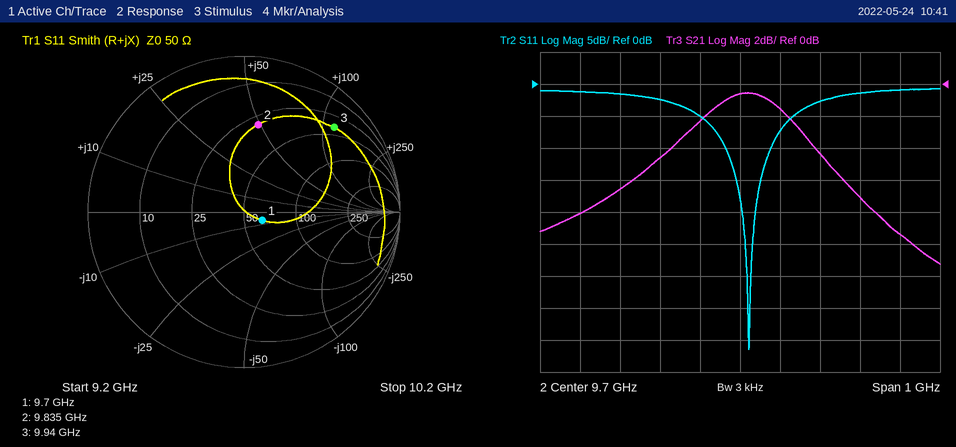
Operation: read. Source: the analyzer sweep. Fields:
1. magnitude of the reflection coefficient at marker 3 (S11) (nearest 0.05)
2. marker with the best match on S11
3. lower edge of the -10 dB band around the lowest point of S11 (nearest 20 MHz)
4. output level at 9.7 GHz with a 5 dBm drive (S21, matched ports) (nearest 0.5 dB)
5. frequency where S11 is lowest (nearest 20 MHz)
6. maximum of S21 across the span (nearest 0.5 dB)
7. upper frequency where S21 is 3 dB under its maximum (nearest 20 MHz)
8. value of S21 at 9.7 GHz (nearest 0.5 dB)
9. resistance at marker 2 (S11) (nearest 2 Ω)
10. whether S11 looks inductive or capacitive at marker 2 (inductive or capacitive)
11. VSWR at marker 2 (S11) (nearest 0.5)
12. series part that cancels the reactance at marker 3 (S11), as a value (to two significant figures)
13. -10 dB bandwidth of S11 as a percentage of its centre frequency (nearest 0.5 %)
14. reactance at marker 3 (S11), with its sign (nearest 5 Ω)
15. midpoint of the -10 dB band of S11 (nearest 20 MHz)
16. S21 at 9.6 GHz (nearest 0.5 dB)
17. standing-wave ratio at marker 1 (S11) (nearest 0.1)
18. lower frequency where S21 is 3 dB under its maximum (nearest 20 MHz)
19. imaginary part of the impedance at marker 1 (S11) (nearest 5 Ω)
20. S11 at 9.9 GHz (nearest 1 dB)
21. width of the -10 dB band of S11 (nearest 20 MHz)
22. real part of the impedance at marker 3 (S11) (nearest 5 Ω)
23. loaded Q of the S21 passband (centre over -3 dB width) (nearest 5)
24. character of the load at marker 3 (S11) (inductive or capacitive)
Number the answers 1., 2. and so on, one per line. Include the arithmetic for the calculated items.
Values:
1. 0.80
2. marker 1
3. 9.66 GHz
4. 5 dBm + (-0.5 dB) = 4.5 dBm
5. 9.72 GHz
6. -0.5 dB
7. 9.88 GHz
8. -0.5 dB
9. 30 Ω
10. inductive
11. 3.5
12. C = 1/(2π × 9.94 GHz × 115 Ω) ≈ 139 fF, so 140 fF to two significant figures
13. 120 MHz / 9.72 GHz ≈ 1.23 %, so 1.0 % to the nearest 0.5 %
14. +115 Ω
15. 9.72 GHz
16. -2.5 dB
17. 1.3
18. 9.54 GHz
19. -5 Ω
20. -3 dB
21. 9.78 GHz − 9.66 GHz = 120 MHz
22. 40 Ω
23. 9.71 GHz / 340 MHz ≈ 28.6, so 30 to the nearest 5
24. inductive
